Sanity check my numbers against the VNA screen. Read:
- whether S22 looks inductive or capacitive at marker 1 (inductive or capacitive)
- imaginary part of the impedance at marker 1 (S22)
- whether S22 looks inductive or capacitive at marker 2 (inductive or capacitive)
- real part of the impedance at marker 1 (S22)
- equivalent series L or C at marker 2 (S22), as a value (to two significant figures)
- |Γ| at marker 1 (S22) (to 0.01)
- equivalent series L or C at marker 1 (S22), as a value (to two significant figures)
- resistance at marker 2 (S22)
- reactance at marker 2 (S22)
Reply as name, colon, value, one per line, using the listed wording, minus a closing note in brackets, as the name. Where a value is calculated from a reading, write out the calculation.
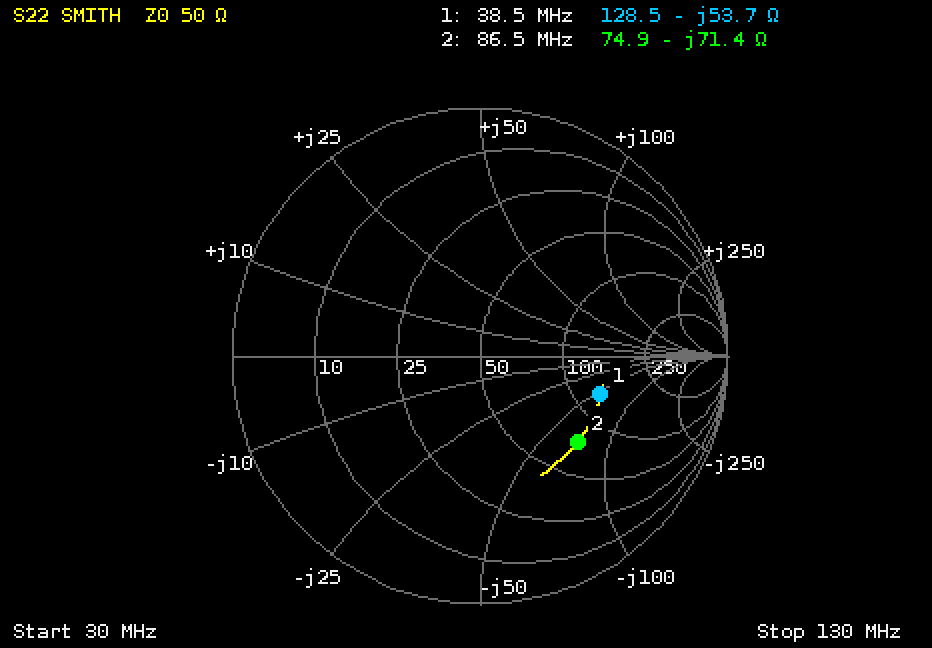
whether S22 looks inductive or capacitive at marker 1: capacitive
imaginary part of the impedance at marker 1: -53.7 Ω
whether S22 looks inductive or capacitive at marker 2: capacitive
real part of the impedance at marker 1: 128.5 Ω
equivalent series L or C at marker 2 (S22), as a value: C = 1/(2π × 86.5 MHz × 71.4 Ω) ≈ 26 pF
|Γ| at marker 1 (S22): 0.51
equivalent series L or C at marker 1 (S22), as a value: C = 1/(2π × 38.5 MHz × 53.7 Ω) ≈ 77 pF
resistance at marker 2: 74.9 Ω
reactance at marker 2: -71.4 Ω
